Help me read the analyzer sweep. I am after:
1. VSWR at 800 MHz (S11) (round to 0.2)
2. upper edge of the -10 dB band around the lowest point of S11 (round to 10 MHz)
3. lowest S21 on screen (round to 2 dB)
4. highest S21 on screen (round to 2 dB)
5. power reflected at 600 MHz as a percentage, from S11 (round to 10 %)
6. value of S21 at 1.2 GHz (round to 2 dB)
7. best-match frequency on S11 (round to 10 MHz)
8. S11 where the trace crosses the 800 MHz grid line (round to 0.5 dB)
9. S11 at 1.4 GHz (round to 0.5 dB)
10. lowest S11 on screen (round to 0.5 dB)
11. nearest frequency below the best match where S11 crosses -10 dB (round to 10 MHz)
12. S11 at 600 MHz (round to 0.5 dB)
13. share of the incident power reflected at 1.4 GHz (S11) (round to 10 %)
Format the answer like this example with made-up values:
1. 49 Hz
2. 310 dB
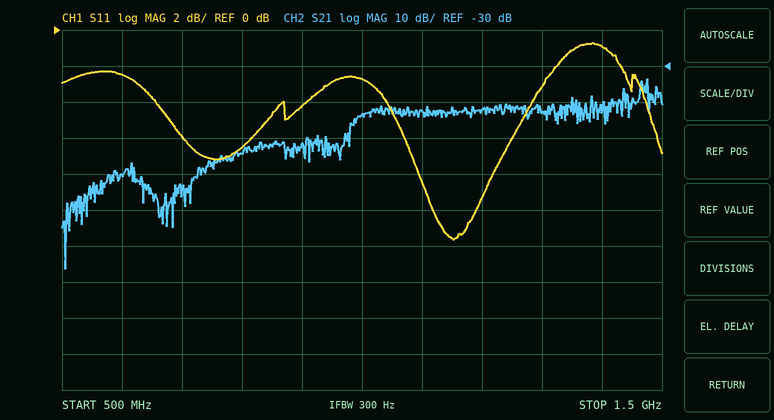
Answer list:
1. 2.8
2. 1.19 GHz
3. -86 dB
4. -34 dB
5. 60 %
6. -42 dB
7. 1.15 GHz
8. -6.5 dB
9. -1.0 dB
10. -11.5 dB
11. 1.12 GHz
12. -2.5 dB
13. 80 %
